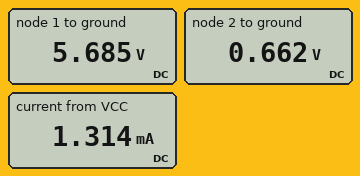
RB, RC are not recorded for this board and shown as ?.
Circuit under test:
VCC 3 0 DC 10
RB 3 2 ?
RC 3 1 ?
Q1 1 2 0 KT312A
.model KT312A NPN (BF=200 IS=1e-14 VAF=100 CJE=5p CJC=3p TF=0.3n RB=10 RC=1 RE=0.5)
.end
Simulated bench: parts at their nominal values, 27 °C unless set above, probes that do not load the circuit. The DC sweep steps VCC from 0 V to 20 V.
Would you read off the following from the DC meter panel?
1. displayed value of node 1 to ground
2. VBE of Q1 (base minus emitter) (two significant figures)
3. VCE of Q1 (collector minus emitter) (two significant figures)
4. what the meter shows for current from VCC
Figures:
5.685 V
660 mV
5.7 V
1.314 mA
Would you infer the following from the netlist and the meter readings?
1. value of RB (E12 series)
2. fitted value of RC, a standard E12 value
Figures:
1.5 MΩ
3.3 kΩ
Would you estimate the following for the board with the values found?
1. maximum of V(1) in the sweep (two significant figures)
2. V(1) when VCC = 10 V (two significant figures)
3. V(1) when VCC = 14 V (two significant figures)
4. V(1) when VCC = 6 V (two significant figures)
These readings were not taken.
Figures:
11 V
5.7 V
7.7 V
3.6 V
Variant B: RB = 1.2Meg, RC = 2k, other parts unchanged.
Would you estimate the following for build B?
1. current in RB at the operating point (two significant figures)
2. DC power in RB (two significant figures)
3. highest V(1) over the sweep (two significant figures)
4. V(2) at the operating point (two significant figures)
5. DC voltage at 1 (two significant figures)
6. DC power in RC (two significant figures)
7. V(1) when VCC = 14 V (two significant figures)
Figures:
7.8 µA
73 µW
13 V
670 mV
6.7 V
5.4 mW
9.2 V
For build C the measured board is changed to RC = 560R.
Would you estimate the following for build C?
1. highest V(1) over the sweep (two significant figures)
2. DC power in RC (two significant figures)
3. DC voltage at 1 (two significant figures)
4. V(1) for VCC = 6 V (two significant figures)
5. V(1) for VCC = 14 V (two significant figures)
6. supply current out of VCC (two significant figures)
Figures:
18 V
1.0 mW
9.2 V
5.6 V
13 V
1.4 mA
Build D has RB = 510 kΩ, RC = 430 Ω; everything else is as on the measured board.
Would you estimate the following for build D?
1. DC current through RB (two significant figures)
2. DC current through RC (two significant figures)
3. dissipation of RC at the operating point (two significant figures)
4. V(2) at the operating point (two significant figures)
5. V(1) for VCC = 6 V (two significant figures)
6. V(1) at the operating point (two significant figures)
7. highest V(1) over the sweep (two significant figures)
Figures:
18 µA
3.9 mA
6.6 mW
690 mV
5.1 V
8.3 V
16 V
